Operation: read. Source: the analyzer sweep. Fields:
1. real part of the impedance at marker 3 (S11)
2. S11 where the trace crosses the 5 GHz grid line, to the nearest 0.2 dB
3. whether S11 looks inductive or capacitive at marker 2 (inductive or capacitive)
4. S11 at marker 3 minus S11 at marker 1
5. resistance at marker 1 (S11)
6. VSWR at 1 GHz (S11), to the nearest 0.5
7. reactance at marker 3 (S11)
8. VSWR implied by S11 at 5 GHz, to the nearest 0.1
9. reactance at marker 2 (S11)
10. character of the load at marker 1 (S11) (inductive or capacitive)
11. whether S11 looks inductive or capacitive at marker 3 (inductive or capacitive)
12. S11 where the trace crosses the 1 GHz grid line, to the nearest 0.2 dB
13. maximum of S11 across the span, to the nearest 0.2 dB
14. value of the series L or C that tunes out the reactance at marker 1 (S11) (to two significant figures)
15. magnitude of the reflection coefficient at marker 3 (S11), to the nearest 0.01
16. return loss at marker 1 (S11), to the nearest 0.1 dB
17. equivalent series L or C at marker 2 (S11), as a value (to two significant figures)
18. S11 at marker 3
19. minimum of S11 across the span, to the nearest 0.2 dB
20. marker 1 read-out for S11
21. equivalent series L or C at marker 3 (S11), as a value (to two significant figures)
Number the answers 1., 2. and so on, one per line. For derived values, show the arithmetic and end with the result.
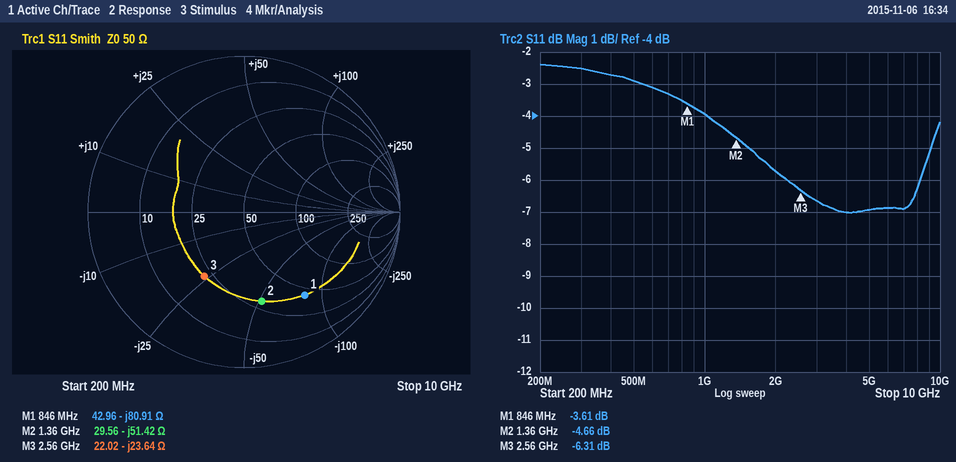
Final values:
1. 22.02 Ω
2. -7.0 dB
3. capacitive
4. -6.31 − (-3.61) = -2.70 dB
5. 42.96 Ω
6. |Γ| = 10^(-4/20) = 0.6310; VSWR = (1 + 0.6310)/(1 − 0.6310) ≈ 4.42, so 4.5 to the nearest 0.5
7. -23.64 Ω
8. |Γ| = 10^(-7/20) = 0.4467; VSWR = (1 + 0.4467)/(1 − 0.4467) ≈ 2.6
9. -51.42 Ω
10. capacitive
11. capacitive
12. -4.0 dB
13. -2.4 dB
14. L = 80.91 Ω/(2π × 846 MHz) ≈ 15 nH
15. 0.48
16. 3.6 dB
17. C = 1/(2π × 1.36 GHz × 51.42 Ω) ≈ 2.3 pF
18. -6.31 dB
19. -7.0 dB
20. -3.61 dB
21. C = 1/(2π × 2.56 GHz × 23.64 Ω) ≈ 2.6 pF
